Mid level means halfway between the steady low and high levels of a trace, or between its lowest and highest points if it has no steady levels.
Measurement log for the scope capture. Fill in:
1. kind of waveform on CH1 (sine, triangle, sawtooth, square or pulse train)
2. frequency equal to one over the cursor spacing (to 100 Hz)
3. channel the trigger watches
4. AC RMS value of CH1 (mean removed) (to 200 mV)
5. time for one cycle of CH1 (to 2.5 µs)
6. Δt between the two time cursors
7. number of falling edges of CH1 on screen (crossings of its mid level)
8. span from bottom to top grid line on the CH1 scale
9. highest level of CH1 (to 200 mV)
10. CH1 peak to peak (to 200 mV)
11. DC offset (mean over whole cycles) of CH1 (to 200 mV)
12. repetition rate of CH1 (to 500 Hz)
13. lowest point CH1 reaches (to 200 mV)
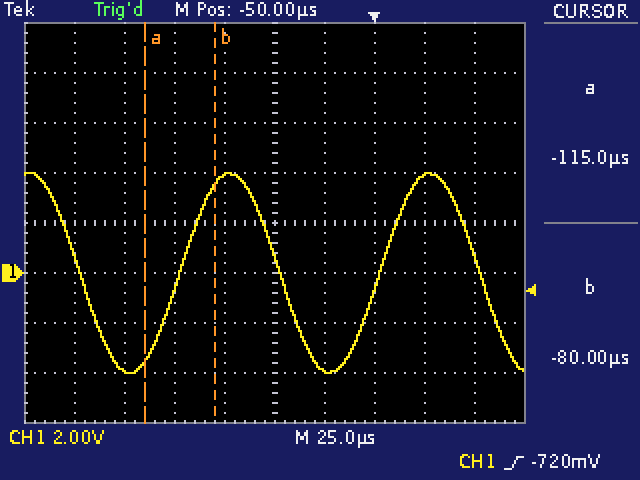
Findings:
sine
28.6 kHz
CH1
2.8 V
100.0 µs
35.0 µs
3
16 V
4.0 V
8.0 V
0.0 V
10.0 kHz
-4.0 V
